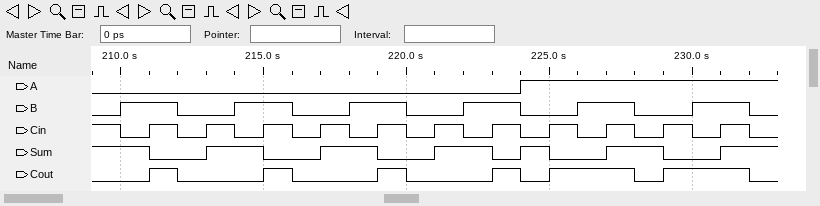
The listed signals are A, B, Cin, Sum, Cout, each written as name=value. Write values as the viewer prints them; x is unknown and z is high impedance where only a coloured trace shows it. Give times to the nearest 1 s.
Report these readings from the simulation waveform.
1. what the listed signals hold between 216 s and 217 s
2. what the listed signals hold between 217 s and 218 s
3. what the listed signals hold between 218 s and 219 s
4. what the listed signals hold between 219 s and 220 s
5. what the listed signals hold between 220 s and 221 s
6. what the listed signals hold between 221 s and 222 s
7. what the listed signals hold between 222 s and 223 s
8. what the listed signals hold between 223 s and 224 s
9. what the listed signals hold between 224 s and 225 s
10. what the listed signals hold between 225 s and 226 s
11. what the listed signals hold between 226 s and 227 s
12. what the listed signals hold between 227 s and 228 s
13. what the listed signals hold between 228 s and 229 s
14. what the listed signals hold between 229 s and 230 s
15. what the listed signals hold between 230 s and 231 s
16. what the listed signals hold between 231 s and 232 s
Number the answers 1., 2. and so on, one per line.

1. A=0, B=0, Cin=0, Sum=0, Cout=0
2. A=0, B=0, Cin=1, Sum=1, Cout=0
3. A=0, B=1, Cin=0, Sum=1, Cout=0
4. A=0, B=1, Cin=1, Sum=0, Cout=1
5. A=0, B=0, Cin=0, Sum=0, Cout=0
6. A=0, B=0, Cin=1, Sum=1, Cout=0
7. A=0, B=1, Cin=0, Sum=1, Cout=0
8. A=0, B=1, Cin=1, Sum=0, Cout=1
9. A=1, B=0, Cin=0, Sum=1, Cout=0
10. A=1, B=0, Cin=1, Sum=0, Cout=1
11. A=1, B=1, Cin=0, Sum=0, Cout=1
12. A=1, B=1, Cin=1, Sum=1, Cout=1
13. A=1, B=0, Cin=0, Sum=1, Cout=0
14. A=1, B=0, Cin=1, Sum=0, Cout=1
15. A=1, B=1, Cin=0, Sum=0, Cout=1
16. A=1, B=1, Cin=1, Sum=1, Cout=1
